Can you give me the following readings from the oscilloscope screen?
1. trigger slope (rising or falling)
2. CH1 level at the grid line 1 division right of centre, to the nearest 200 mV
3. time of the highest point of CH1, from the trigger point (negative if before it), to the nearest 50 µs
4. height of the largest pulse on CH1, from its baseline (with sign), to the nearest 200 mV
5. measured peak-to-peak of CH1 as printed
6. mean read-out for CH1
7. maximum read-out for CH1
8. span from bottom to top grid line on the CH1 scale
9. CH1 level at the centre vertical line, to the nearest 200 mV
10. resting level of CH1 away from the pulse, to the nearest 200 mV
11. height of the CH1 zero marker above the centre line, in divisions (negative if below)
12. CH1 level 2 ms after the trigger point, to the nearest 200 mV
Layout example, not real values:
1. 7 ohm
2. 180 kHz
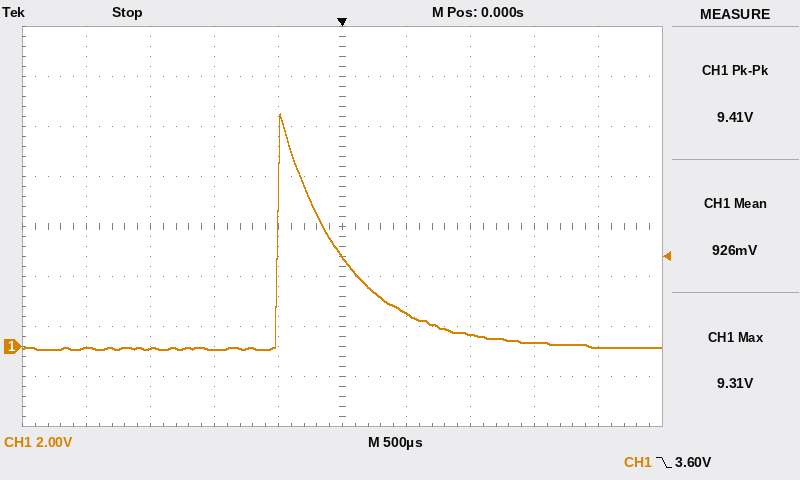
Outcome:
1. falling
2. 1.4 V
3. -500 µs
4. +9.4 V
5. 9.41 V
6. 926 mV
7. 9.31 V
8. 16 V
9. 3.6 V
10. 0.0 V
11. -2.4 div
12. 0.0 V
